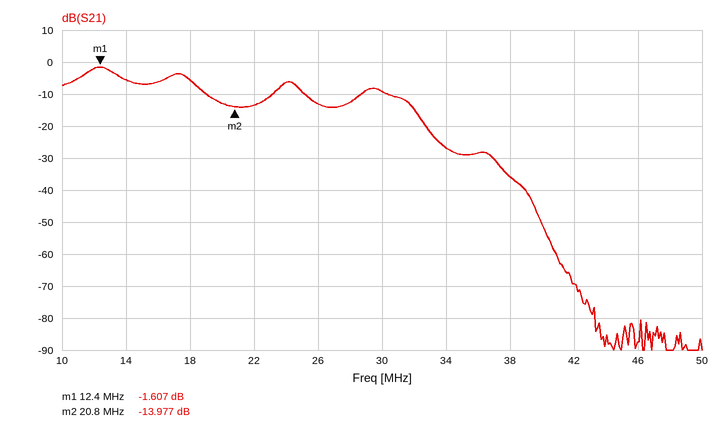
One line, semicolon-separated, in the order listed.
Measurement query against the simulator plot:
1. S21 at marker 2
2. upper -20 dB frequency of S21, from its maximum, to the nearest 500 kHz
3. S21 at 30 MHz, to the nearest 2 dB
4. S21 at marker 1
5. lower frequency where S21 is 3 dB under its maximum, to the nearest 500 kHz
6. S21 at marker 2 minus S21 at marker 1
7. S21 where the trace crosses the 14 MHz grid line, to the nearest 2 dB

-13.977 dB; 33.0 MHz; -10 dB; -1.607 dB; 11.0 MHz; -12.370 dB; -6 dB
